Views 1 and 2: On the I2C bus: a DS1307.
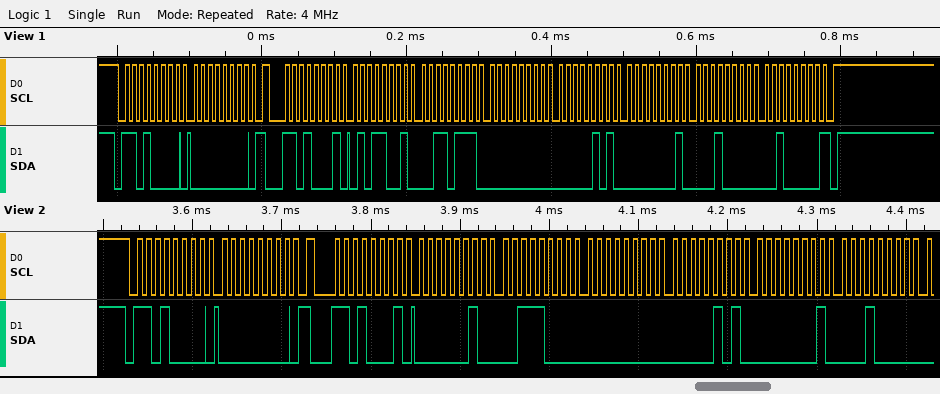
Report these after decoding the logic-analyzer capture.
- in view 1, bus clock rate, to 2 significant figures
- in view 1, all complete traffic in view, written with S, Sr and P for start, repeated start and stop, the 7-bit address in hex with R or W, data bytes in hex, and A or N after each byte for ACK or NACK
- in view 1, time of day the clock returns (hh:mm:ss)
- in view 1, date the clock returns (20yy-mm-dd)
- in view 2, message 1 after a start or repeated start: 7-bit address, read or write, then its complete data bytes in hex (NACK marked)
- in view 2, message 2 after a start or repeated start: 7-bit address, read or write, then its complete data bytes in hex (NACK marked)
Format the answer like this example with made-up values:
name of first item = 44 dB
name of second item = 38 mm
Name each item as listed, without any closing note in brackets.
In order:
in view 1, bus clock rate, to 2 significant figures = 100 kHz
in view 1, all complete traffic in view, written with S, Sr and P for start, repeated start and stop, the 7-bit address in hex with R or W, data bytes in hex, and A or N after each byte for ACK or NACK = S 68W A 00 A Sr 68R A 59 A 37 A 00 A 05 A 01 A 10 A 20 N P
in view 1, time of day the clock returns = 00:37:59
in view 1, date the clock returns = 2020-10-01
in view 2, message 1 after a start or repeated start: 7-bit address, read or write, then its complete data bytes in hex = 0x68 write: 00
in view 2, message 2 after a start or repeated start: 7-bit address, read or write, then its complete data bytes in hex = 0x68 read: 02 38 00 05 01 10
